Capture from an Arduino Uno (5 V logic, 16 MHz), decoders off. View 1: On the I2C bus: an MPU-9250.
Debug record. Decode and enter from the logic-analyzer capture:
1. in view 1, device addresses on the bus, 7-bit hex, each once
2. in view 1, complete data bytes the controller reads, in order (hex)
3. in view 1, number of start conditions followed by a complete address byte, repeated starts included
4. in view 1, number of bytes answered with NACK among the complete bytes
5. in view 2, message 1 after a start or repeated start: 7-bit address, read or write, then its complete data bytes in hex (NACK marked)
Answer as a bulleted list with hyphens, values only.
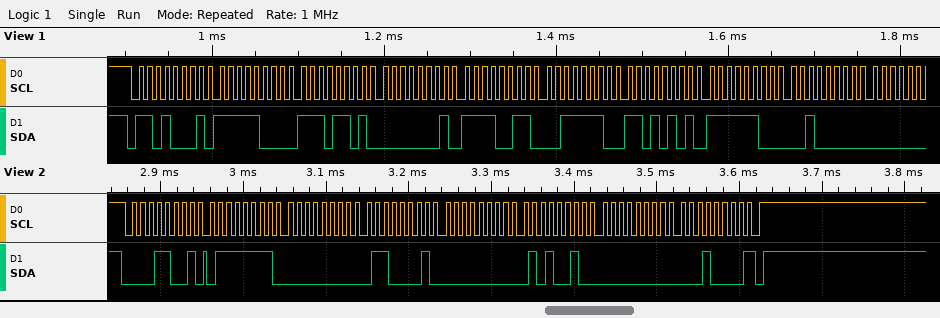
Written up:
- 0x68
- F8 ED 01 F3 3E D5 FC 20
- 1
- 0
- 0x0C read: 7F 00 61 00 52 00 10 NACK
